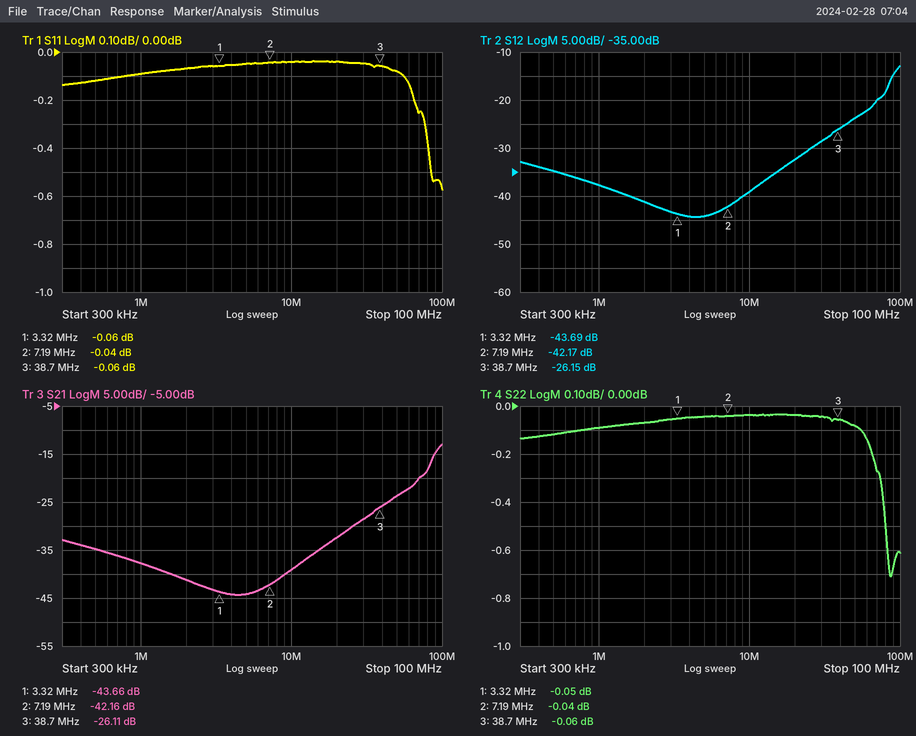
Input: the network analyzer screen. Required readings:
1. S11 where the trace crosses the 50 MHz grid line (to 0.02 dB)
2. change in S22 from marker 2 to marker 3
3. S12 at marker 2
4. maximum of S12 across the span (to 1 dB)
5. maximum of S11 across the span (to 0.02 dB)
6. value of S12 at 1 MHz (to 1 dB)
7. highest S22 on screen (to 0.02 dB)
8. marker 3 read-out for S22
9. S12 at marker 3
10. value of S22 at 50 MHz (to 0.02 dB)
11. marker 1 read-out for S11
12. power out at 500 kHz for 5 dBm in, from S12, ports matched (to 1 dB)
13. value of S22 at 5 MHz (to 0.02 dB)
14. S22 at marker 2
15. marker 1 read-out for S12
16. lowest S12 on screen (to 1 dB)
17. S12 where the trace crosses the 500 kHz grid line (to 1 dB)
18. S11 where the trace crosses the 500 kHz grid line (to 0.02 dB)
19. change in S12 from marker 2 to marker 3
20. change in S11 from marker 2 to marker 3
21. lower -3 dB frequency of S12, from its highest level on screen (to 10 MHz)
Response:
-0.08 dB
-0.02 dB
-42.17 dB
-13 dB
-0.04 dB
-38 dB
-0.04 dB
-0.06 dB
-26.15 dB
-0.08 dB
-0.06 dB
-30 dBm
-0.04 dB
-0.04 dB
-43.69 dB
-44 dB
-35 dB
-0.12 dB
16.02 dB
-0.02 dB
90 MHz
